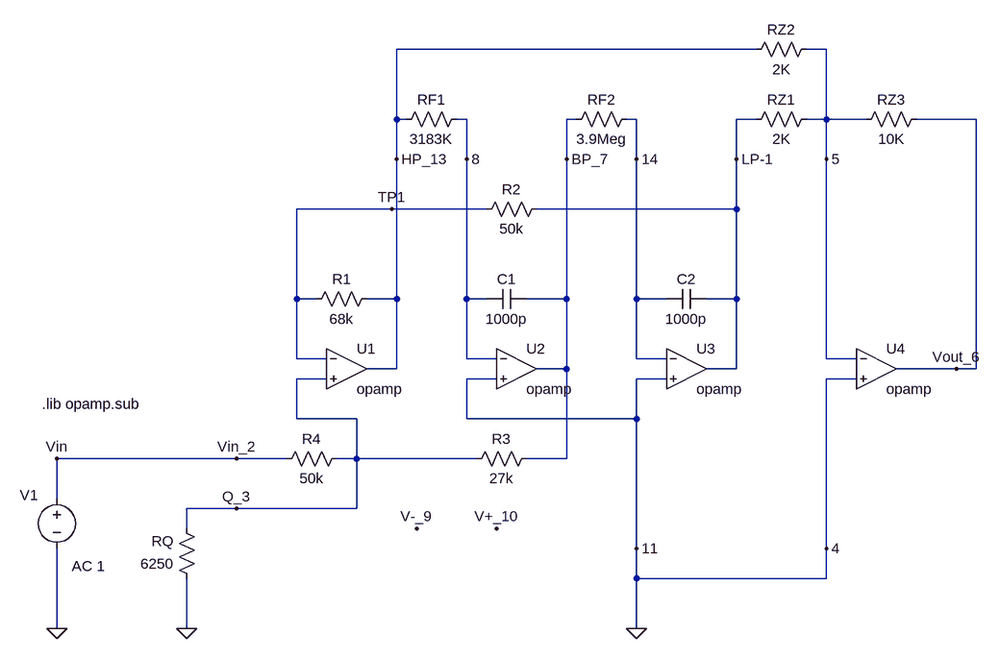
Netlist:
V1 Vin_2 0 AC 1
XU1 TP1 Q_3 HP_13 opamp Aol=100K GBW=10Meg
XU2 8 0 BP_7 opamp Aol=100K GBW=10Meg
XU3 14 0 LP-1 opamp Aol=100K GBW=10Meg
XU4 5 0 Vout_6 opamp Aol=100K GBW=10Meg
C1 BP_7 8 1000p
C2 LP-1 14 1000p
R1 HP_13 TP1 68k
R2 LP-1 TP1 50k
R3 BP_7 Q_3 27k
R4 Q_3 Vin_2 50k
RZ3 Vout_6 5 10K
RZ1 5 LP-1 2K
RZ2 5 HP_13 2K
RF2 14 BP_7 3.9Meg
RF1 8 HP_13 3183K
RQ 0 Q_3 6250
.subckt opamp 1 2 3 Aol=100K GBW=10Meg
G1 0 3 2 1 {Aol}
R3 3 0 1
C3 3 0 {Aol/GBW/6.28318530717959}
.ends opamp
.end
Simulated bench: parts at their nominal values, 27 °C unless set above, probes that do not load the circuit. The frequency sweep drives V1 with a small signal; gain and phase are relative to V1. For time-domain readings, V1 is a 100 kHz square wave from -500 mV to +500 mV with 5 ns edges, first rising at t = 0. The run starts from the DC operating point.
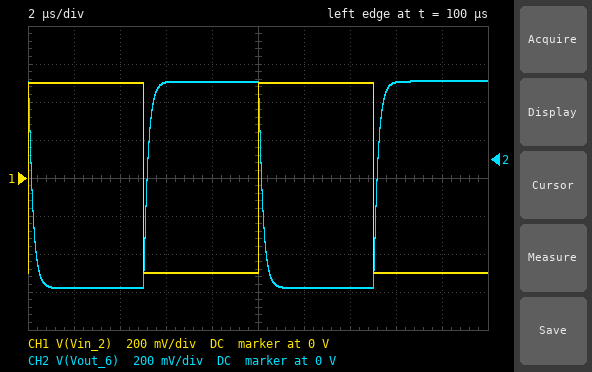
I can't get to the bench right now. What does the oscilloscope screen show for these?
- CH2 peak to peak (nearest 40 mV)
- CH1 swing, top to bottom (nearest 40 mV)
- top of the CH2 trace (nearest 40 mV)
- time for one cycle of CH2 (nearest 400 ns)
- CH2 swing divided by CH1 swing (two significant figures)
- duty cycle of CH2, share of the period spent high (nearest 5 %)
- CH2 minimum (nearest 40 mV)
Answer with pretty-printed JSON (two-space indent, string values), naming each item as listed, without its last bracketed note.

{
  "CH2 peak to peak": "1.08 V",
  "CH1 swing, top to bottom": "1.00 V",
  "top of the CH2 trace": "400 mV",
  "time for one cycle of CH2": "10.0 µs",
  "CH2 swing divided by CH1 swing": "1.1",
  "duty cycle of CH2, share of the period spent high": "50 %",
  "CH2 minimum": "-680 mV"
}
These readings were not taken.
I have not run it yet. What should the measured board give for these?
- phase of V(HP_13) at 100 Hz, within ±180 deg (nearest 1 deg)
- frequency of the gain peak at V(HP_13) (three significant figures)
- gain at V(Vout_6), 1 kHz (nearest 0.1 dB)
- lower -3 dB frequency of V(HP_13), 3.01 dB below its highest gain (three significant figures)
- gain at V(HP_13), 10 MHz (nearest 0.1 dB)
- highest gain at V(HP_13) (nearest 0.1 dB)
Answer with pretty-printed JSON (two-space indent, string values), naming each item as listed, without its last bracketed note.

{
  "phase of V(HP_13) at 100 Hz, within ±180 deg": "16 deg",
  "frequency of the gain peak at V(HP_13)": "54.7 Hz",
  "gain at V(Vout_6), 1 kHz": "0.7 dB",
  "lower -3 dB frequency of V(HP_13), 3.01 dB below its highest gain": "46.2 Hz",
  "gain at V(HP_13), 10 MHz": "-21.4 dB",
  "highest gain at V(HP_13)": "-4.7 dB"
}
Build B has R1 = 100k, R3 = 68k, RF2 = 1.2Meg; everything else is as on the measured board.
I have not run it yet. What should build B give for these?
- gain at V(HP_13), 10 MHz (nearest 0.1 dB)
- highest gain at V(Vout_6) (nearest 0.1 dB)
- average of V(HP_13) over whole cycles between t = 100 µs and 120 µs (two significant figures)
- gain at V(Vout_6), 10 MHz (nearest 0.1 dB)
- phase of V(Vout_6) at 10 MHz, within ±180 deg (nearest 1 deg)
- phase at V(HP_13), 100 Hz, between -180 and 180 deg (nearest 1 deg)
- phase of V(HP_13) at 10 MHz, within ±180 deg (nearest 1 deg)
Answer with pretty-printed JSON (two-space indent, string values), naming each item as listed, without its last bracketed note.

{
  "gain at V(HP_13), 10 MHz": "-20.2 dB",
  "highest gain at V(Vout_6)": "18.0 dB",
  "average of V(HP_13) over whole cycles between t = 100 µs and 120 µs": "150 mV",
  "gain at V(Vout_6), 10 MHz": "-27.1 dB",
  "phase of V(Vout_6) at 10 MHz, within ±180 deg": "24 deg",
  "phase at V(HP_13), 100 Hz, between -180 and 180 deg": "161 deg",
  "phase of V(HP_13) at 10 MHz, within ±180 deg": "-72 deg"
}
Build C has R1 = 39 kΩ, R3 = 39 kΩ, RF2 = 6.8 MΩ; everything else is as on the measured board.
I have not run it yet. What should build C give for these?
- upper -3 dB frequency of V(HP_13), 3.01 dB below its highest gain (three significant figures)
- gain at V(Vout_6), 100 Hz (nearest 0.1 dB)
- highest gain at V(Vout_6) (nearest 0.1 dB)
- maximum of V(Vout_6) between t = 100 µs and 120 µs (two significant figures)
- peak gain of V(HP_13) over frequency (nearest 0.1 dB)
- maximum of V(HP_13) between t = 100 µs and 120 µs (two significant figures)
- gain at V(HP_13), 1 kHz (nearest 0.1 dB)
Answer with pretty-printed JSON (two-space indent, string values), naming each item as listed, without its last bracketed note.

{
  "upper -3 dB frequency of V(HP_13), 3.01 dB below its highest gain": "40.0 Hz",
  "gain at V(Vout_6), 100 Hz": "-1.6 dB",
  "highest gain at V(Vout_6)": "1.6 dB",
  "maximum of V(Vout_6) between t = 100 µs and 120 µs": "560 mV",
  "peak gain of V(HP_13) over frequency": "-6.4 dB",
  "maximum of V(HP_13) between t = 100 µs and 120 µs": "170 mV",
  "gain at V(HP_13), 1 kHz": "-15.2 dB"
}
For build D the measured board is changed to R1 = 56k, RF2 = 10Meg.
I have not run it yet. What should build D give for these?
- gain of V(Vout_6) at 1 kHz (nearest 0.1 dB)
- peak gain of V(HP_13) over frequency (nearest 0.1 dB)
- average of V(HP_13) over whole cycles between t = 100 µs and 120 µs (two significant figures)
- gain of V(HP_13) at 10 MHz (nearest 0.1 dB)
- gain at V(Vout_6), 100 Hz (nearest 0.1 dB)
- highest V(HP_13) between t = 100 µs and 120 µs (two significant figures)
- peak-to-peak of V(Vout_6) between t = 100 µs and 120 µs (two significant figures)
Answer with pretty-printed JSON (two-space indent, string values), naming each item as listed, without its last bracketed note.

{
  "gain of V(Vout_6) at 1 kHz": "-0.2 dB",
  "peak gain of V(HP_13) over frequency": "-9.4 dB",
  "average of V(HP_13) over whole cycles between t = 100 µs and 120 µs": "96 mV",
  "gain of V(HP_13) at 10 MHz": "-21.6 dB",
  "gain at V(Vout_6), 100 Hz": "-0.3 dB",
  "highest V(HP_13) between t = 100 µs and 120 µs": "190 mV",
  "peak-to-peak of V(Vout_6) between t = 100 µs and 120 µs": "980 mV"
}
